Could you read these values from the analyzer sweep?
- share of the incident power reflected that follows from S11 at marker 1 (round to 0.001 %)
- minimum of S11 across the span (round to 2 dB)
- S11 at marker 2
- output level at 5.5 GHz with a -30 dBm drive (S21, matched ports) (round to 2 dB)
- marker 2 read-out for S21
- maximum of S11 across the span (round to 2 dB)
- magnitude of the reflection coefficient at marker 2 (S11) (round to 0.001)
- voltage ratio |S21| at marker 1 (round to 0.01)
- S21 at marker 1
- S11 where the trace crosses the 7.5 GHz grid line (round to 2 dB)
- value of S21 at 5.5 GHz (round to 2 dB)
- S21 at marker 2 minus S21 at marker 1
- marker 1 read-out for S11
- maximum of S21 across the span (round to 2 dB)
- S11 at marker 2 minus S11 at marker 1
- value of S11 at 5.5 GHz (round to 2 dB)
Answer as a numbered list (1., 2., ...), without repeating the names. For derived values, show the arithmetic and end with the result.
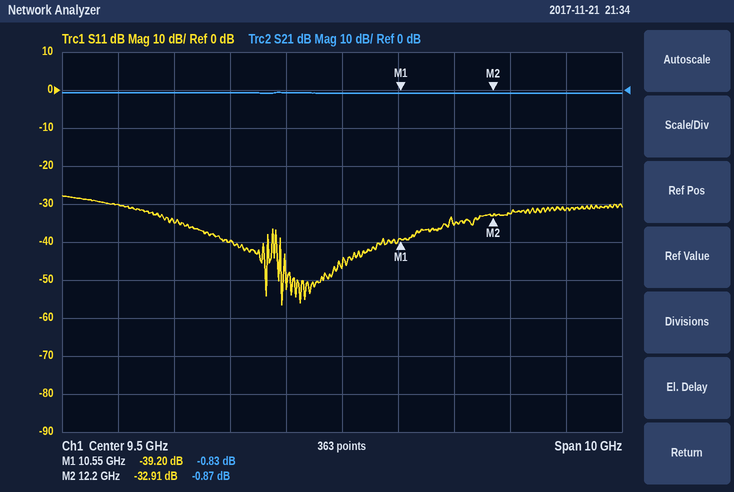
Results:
1. 10^(-39.2/10) ≈ 0.012 %
2. -56 dB
3. -32.91 dB
4. -30 dBm + (0 dB) = -30 dBm
5. -0.87 dB
6. -28 dB
7. 10^(-32.91/20) ≈ 0.023
8. 10^(-0.83/20) ≈ 0.91
9. -0.83 dB
10. -40 dB
11. 0 dB
12. -0.87 − (-0.83) = -0.04 dB
13. -39.20 dB
14. 0 dB
15. -32.91 − (-39.2) = 6.29 dB
16. -30 dB
